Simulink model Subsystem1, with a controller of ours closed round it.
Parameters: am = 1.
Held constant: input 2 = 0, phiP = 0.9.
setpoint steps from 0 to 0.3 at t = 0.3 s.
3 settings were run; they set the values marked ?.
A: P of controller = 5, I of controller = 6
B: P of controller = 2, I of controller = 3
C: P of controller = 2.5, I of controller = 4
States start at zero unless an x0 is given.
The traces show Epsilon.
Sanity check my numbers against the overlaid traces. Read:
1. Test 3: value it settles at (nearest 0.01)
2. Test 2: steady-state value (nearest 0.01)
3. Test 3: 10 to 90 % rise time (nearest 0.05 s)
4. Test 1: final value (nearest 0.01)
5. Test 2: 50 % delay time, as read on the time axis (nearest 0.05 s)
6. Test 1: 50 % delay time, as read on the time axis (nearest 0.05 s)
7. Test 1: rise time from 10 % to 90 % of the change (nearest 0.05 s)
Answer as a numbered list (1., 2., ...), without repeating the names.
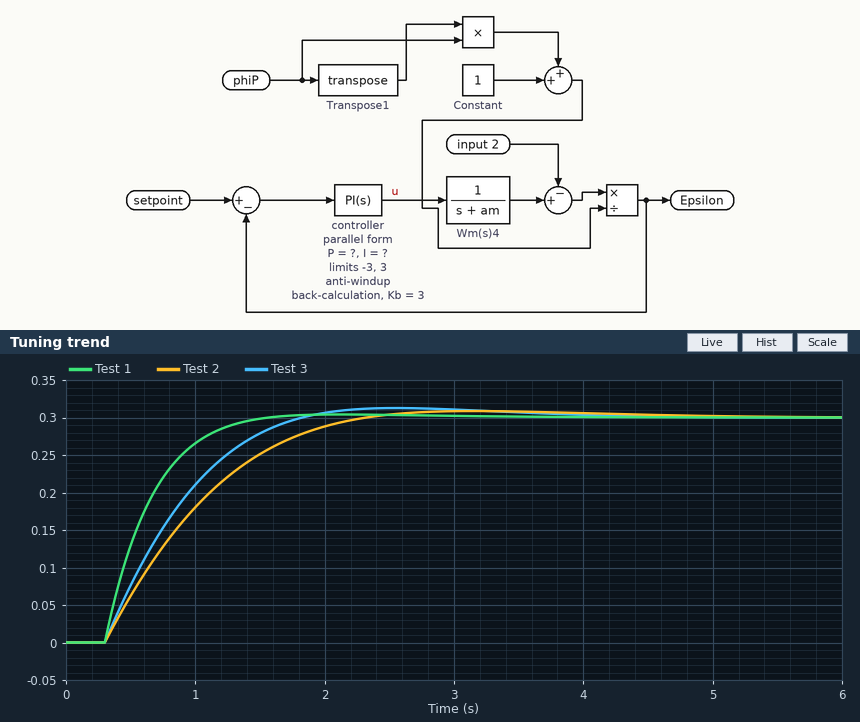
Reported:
1. 0.30
2. 0.30
3. 1.05 s
4. 0.30
5. 0.85 s
6. 0.55 s
7. 0.70 s
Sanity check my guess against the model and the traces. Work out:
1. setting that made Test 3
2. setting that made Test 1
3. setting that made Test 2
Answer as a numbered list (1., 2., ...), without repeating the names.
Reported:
1. C
2. A
3. B
